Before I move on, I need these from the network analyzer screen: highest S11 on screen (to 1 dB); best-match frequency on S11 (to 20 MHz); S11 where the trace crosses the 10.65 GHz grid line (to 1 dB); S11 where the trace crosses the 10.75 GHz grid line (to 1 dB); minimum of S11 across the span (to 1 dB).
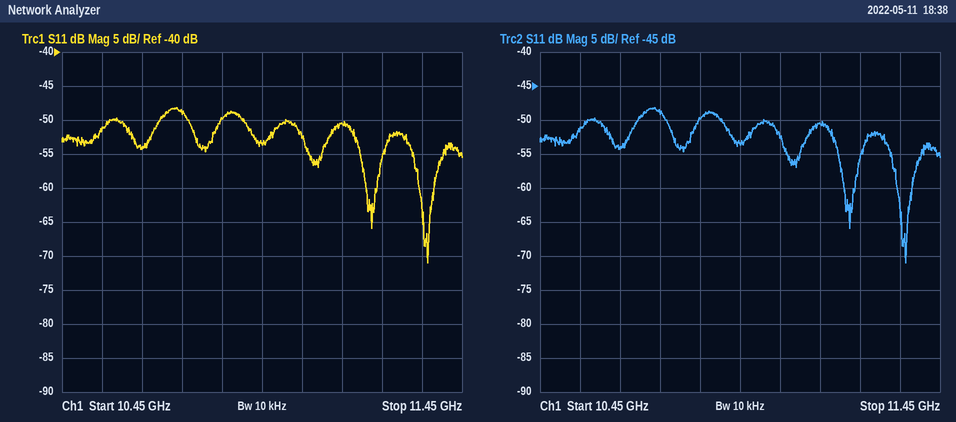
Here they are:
-48 dB
11.36 GHz
-54 dB
-49 dB
-71 dB
